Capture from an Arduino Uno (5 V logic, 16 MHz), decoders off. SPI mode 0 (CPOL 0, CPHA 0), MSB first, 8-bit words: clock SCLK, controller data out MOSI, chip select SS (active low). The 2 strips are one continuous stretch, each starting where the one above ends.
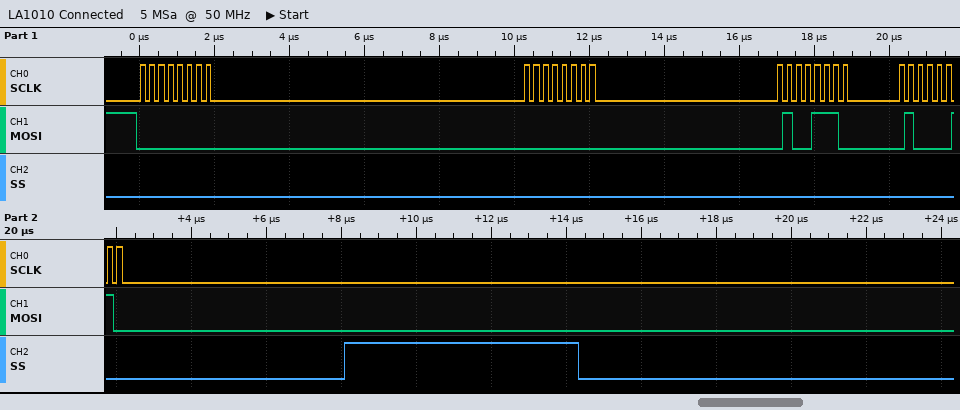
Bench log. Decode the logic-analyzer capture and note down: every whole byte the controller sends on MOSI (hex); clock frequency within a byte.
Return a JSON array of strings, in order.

["00 00 4E 42", "4 MHz"]
